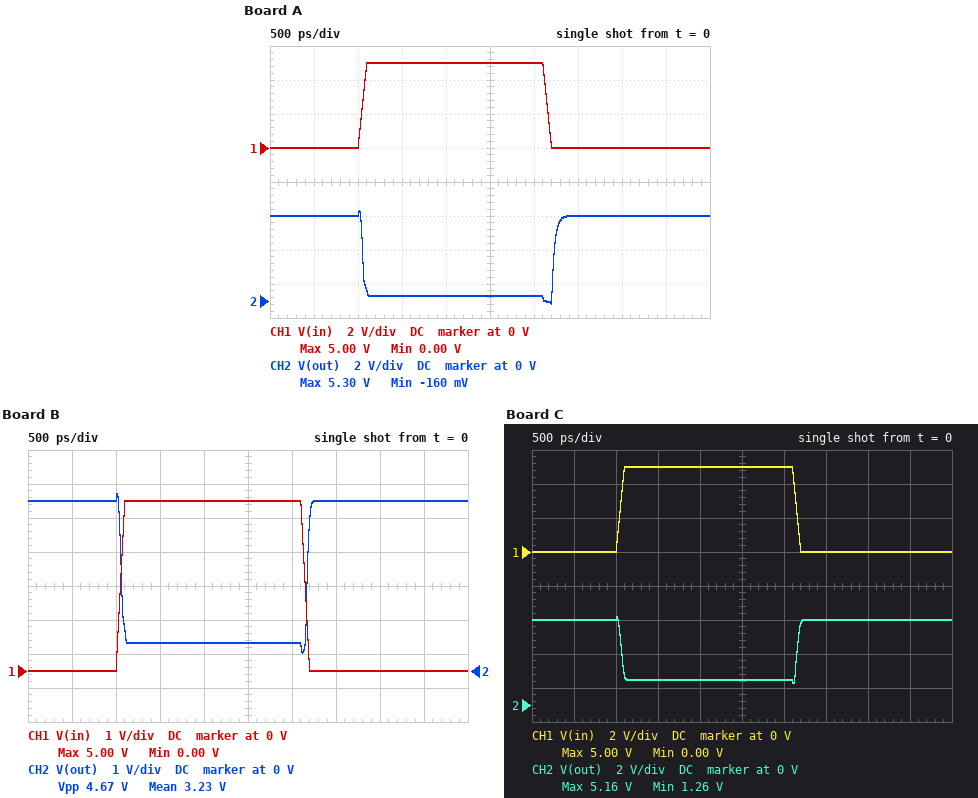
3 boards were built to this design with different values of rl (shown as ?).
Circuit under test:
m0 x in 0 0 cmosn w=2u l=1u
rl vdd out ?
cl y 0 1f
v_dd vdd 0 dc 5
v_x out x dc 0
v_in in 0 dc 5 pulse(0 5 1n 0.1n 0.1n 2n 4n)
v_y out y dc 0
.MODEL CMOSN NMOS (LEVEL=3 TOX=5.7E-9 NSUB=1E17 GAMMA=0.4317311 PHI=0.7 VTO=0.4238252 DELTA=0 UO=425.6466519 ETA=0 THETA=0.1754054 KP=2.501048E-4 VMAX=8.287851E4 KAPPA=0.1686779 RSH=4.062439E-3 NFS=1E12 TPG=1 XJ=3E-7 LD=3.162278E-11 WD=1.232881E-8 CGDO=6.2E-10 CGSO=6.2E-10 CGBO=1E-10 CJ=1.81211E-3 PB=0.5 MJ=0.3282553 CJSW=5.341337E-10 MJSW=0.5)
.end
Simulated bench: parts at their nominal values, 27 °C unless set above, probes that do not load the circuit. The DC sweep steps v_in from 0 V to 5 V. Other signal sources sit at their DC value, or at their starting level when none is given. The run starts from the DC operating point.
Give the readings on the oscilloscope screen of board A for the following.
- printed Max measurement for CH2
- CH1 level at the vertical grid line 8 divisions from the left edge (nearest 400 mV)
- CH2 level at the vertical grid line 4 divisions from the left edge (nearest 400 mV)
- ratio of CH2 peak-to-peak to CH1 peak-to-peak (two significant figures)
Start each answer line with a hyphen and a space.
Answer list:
- 5.30 V
- 0 V
- 400 mV
- 1.1
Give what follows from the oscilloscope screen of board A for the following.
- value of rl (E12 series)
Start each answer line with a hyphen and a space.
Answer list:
- 15 kΩ
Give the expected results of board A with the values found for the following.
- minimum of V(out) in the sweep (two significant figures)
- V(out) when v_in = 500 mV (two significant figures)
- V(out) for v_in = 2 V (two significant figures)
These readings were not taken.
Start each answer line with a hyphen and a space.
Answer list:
- 280 mV
- 5.0 V
- 850 mV
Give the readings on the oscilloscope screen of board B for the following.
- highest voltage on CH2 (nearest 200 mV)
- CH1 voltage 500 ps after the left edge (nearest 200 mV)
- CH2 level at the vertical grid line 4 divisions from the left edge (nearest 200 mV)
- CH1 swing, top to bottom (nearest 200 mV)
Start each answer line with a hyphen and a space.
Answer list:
- 5.2 V
- 0 V
- 800 mV
- 5.0 V
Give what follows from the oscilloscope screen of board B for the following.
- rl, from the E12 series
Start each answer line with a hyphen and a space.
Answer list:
- 5.6 kΩ
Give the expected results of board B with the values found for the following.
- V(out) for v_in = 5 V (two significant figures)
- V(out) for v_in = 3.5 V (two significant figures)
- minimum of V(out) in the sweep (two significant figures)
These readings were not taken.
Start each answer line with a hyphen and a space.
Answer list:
- 810 mV
- 1.2 V
- 810 mV
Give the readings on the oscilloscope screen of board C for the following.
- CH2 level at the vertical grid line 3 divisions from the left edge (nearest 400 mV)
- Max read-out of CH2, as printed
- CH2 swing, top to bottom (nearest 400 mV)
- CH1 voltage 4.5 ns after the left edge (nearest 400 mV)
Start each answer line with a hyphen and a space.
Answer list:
- 1.6 V
- 5.16 V
- 4.0 V
- 0 V
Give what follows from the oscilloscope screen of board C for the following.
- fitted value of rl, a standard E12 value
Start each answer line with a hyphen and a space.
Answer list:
- 3.3 kΩ
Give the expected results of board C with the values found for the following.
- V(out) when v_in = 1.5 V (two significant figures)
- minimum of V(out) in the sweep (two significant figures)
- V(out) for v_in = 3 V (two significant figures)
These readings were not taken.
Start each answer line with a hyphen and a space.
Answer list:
- 4.4 V
- 1.5 V
- 3.0 V
